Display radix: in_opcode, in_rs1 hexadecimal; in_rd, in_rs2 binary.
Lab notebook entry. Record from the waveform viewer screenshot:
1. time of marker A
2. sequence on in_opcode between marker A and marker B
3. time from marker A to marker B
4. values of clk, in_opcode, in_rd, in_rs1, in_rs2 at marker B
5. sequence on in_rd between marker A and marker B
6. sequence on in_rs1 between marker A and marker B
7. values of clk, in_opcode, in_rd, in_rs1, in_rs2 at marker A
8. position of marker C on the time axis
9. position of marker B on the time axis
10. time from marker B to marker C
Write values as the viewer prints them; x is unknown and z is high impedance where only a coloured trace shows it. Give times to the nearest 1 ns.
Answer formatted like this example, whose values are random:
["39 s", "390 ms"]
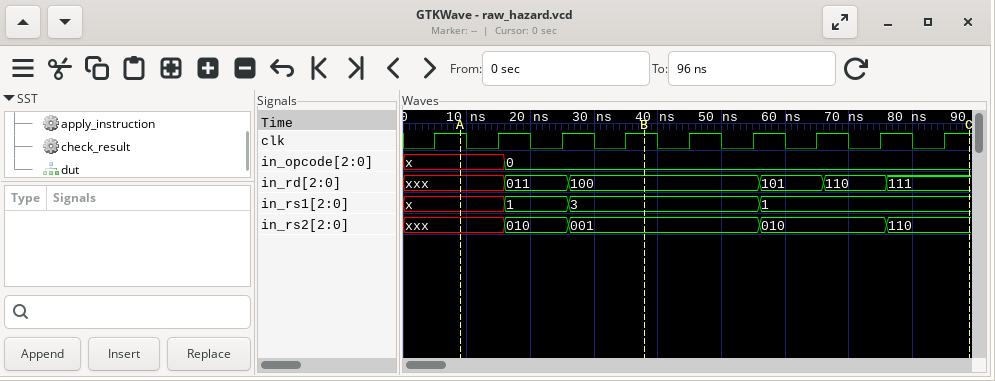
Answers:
["9 ns", "x, 0", "29 ns", "clk=1, in_opcode=0, in_rd=100, in_rs1=3, in_rs2=001", "xxx, 011, 100", "x, 1, 3", "clk=1, in_opcode=x, in_rd=xxx, in_rs1=x, in_rs2=xxx", "89 ns", "38 ns", "51 ns"]
